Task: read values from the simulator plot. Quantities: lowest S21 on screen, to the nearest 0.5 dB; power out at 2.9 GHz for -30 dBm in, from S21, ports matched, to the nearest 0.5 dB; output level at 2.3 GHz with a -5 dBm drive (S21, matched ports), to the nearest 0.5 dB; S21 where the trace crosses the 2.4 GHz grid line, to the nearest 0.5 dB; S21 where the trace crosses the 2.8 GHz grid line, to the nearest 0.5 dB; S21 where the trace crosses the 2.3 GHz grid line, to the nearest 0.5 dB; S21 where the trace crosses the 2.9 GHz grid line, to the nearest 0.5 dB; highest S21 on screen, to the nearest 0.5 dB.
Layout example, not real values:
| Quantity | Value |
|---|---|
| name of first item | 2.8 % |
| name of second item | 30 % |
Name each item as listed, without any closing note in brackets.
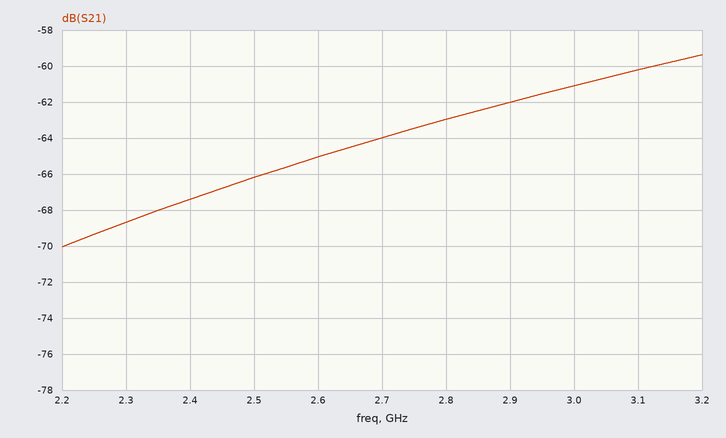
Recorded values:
| Quantity | Value |
|---|---|
| lowest S21 on screen, to the nearest 0.5 dB | -70.0 dB |
| power out at 2.9 GHz for -30 dBm in, from S21, ports matched, to the nearest 0.5 dB | -92.0 dBm |
| output level at 2.3 GHz with a -5 dBm drive (S21, matched ports), to the nearest 0.5 dB | -73.5 dBm |
| S21 where the trace crosses the 2.4 GHz grid line, to the nearest 0.5 dB | -67.5 dB |
| S21 where the trace crosses the 2.8 GHz grid line, to the nearest 0.5 dB | -63.0 dB |
| S21 where the trace crosses the 2.3 GHz grid line, to the nearest 0.5 dB | -68.5 dB |
| S21 where the trace crosses the 2.9 GHz grid line, to the nearest 0.5 dB | -62.0 dB |
| highest S21 on screen, to the nearest 0.5 dB | -59.5 dB |
